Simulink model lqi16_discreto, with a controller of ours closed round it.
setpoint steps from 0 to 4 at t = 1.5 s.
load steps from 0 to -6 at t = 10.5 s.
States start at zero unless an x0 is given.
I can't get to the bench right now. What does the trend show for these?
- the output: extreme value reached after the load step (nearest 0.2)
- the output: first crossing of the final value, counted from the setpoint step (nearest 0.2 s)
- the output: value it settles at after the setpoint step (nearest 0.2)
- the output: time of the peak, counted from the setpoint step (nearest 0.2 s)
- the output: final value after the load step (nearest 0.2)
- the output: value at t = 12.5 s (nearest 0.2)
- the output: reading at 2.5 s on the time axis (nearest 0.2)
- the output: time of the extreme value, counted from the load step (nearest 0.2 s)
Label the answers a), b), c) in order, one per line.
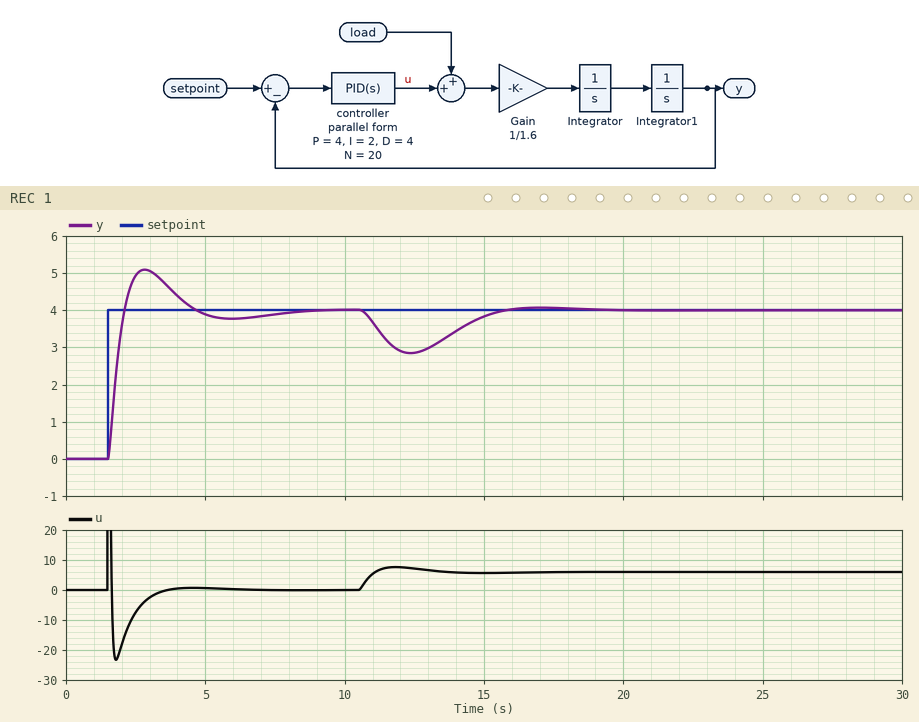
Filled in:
a) 2.8
b) 0.6 s
c) 4.0
d) 1.4 s
e) 4.0
f) 2.8
g) 5.0
h) 1.8 s
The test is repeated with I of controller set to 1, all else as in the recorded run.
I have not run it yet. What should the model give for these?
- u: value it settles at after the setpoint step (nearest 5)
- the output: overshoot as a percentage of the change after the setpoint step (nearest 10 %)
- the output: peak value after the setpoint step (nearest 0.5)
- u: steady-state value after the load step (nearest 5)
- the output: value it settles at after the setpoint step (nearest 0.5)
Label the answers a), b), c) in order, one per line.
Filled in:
a) 0
b) 20 %
c) 5.0
d) 5
e) 4.0
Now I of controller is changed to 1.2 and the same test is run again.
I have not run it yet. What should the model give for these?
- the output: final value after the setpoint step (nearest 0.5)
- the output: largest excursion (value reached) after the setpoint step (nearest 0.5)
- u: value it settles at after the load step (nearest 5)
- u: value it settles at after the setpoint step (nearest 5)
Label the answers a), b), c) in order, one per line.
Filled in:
a) 4.0
b) 5.0
c) 5
d) 0
